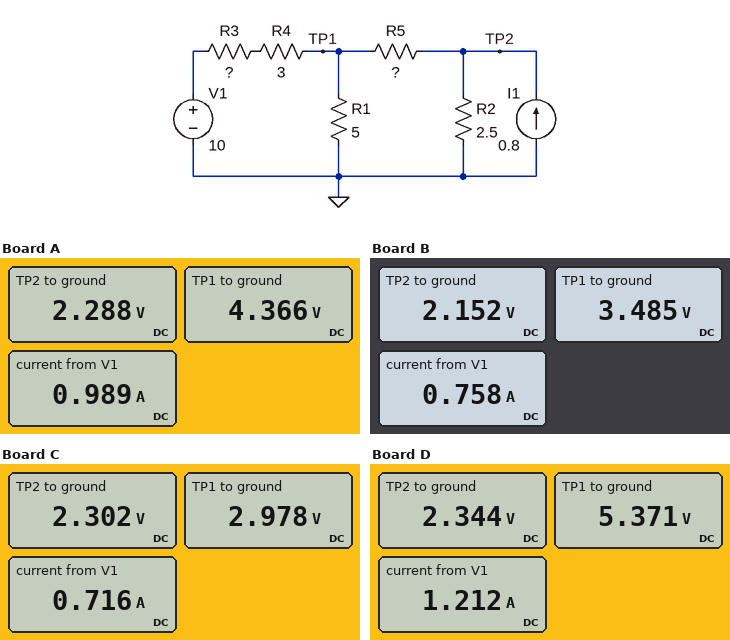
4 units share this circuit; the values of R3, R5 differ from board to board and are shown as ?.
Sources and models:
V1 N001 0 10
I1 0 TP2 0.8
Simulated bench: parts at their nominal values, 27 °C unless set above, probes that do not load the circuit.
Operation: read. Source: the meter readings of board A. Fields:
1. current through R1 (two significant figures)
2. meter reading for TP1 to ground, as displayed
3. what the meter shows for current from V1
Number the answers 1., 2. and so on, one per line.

1. 870 mA
2. 4.366 V
3. 0.989 A
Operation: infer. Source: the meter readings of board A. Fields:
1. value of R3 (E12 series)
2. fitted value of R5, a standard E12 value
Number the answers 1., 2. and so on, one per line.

1. 2.7 Ω
2. 18 Ω
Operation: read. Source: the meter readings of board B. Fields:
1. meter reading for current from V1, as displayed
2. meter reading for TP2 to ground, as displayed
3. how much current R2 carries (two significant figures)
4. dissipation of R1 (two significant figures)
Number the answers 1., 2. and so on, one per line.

1. 0.758 A
2. 2.152 V
3. 860 mA
4. 2.4 W
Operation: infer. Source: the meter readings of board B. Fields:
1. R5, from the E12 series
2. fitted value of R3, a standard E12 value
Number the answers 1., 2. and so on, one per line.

1. 22 Ω
2. 5.6 Ω
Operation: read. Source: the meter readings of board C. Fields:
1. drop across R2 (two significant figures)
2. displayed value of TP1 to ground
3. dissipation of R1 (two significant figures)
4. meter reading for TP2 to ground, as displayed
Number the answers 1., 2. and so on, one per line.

1. 2.3 V
2. 2.978 V
3. 1.8 W
4. 2.302 V
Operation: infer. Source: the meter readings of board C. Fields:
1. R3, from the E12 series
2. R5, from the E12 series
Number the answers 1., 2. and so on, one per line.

1. 6.8 Ω
2. 5.6 Ω
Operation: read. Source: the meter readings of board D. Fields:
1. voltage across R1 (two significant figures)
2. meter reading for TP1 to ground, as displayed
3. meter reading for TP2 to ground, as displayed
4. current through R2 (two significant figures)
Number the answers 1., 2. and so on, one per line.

1. 5.4 V
2. 5.371 V
3. 2.344 V
4. 940 mA
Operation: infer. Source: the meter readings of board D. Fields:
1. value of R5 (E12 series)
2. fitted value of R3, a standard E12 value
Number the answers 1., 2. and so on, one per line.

1. 22 Ω
2. 0.82 Ω
